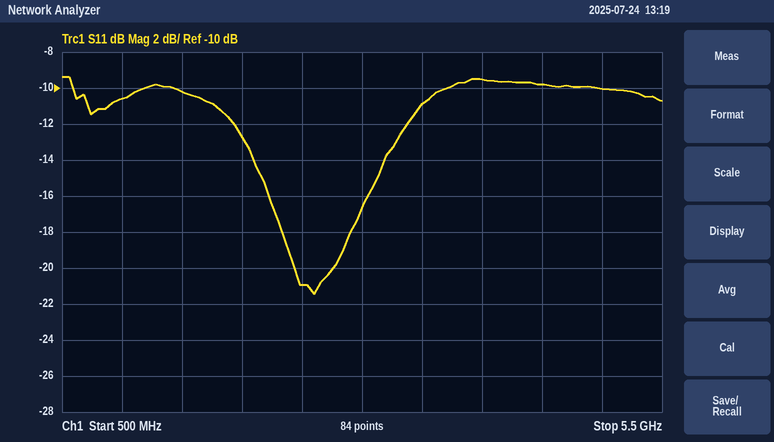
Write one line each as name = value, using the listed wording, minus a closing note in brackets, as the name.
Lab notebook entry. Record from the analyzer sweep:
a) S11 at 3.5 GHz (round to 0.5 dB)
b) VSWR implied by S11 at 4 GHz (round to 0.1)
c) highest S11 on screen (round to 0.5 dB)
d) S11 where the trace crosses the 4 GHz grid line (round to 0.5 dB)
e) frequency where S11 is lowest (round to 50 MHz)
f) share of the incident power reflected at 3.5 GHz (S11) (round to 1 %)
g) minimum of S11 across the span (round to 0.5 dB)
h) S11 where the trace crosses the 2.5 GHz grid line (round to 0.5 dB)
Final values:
S11 at 3.5 GHz = -11.0 dB
VSWR implied by S11 at 4 GHz = 2.0
highest S11 on screen = -9.5 dB
S11 where the trace crosses the 4 GHz grid line = -9.5 dB
frequency where S11 is lowest = 2.60 GHz
share of the incident power reflected at 3.5 GHz (S11) = 8 %
minimum of S11 across the span = -21.5 dB
S11 where the trace crosses the 2.5 GHz grid line = -21.0 dB
